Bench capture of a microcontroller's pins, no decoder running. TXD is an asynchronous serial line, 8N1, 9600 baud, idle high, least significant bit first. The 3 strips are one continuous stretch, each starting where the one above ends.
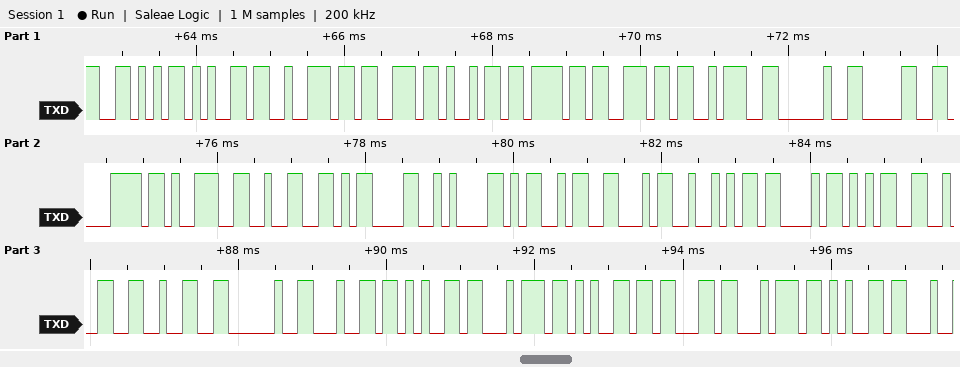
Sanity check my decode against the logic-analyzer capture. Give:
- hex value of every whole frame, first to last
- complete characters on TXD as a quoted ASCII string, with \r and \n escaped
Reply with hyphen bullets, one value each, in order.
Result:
- 56 65 72 73 69 6F 6E 3A 20 30 78 39 32 0D 0A 4D 46 52 43 35 32 32 20 64 65 74 65 63 74 65
- "Version: 0x92\r\nMFRC522 detecte"
